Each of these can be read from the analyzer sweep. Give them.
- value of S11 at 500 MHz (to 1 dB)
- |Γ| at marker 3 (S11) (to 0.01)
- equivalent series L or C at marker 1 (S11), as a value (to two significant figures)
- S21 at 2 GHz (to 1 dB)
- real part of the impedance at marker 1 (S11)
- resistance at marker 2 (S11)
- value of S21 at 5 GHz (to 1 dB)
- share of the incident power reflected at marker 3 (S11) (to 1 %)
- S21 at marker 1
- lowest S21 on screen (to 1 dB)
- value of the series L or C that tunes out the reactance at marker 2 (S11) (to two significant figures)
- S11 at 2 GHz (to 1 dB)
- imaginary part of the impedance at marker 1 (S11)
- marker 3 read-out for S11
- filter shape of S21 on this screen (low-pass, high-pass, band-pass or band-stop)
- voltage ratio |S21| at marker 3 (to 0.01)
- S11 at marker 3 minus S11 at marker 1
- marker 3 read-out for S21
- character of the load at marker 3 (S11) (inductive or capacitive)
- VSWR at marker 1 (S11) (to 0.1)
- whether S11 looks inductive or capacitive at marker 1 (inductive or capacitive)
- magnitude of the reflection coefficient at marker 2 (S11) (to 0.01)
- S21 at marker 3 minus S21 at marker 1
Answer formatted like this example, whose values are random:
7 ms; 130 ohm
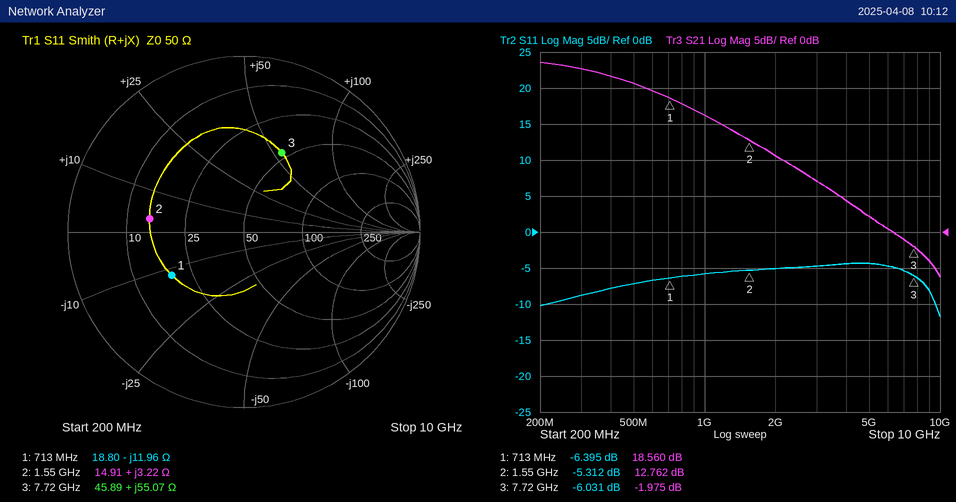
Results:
-7 dB; 0.50; 19 pF; 11 dB; 18.80 Ω; 14.91 Ω; 2 dB; 25 %; 18.560 dB; -6 dB; 32 pF; -5 dB; -11.96 Ω; -6.031 dB; low-pass; 0.80; 0.364 dB; -1.975 dB; inductive; 2.8; capacitive; 0.54; -20.535 dB
